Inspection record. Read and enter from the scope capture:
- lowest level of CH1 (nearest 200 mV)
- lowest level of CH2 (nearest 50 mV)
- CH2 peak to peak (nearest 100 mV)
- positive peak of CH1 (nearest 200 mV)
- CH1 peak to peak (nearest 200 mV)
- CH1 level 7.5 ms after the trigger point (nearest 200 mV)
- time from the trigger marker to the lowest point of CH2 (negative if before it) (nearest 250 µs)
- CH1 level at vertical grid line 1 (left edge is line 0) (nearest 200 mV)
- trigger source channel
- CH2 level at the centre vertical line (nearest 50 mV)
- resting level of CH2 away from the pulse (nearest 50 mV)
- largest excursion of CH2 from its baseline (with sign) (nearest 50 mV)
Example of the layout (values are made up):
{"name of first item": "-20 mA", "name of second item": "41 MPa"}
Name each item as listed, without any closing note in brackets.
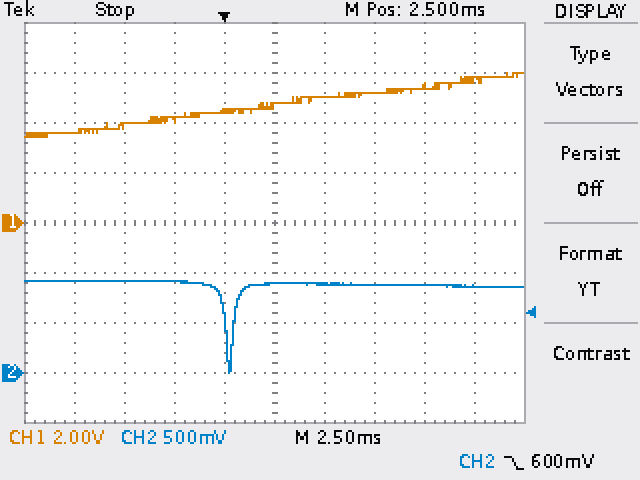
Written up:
{"lowest level of CH1": "3.4 V", "lowest level of CH2": "0 mV", "CH2 peak to peak": "900 mV", "positive peak of CH1": "6.0 V", "CH1 peak to peak": "2.6 V", "CH1 level 7.5 ms after the trigger point": "5.2 V", "time from the trigger marker to the lowest point of CH2 (negative if before it)": "+250 µs", "CH1 level at vertical grid line 1 (left edge is line 0)": "3.6 V", "trigger source channel": "CH2", "CH2 level at the centre vertical line": "900 mV", "resting level of CH2 away from the pulse": "900 mV", "largest excursion of CH2 from its baseline (with sign)": "-900 mV"}
